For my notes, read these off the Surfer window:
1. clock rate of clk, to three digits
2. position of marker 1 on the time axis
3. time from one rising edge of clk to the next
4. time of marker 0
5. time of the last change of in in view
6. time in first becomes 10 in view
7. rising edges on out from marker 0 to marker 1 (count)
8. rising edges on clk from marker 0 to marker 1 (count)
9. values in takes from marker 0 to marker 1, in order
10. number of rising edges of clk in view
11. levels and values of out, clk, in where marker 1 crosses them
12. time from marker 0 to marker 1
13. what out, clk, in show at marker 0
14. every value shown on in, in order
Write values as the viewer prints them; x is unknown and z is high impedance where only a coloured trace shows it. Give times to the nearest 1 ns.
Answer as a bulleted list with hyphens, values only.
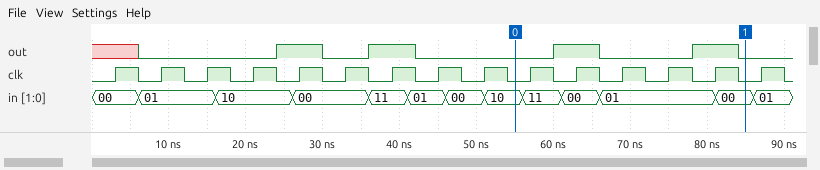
- 167 MHz
- 85 ns
- 6 ns
- 55 ns
- 86 ns
- 16 ns
- 2
- 5
- 10, 11, 00, 01, 00
- 15
- out=0, clk=0, in=00
- 30 ns
- out=0, clk=0, in=10
- 00, 01, 10, 00, 11, 01, 00, 10, 11, 00, 01, 00, 01
